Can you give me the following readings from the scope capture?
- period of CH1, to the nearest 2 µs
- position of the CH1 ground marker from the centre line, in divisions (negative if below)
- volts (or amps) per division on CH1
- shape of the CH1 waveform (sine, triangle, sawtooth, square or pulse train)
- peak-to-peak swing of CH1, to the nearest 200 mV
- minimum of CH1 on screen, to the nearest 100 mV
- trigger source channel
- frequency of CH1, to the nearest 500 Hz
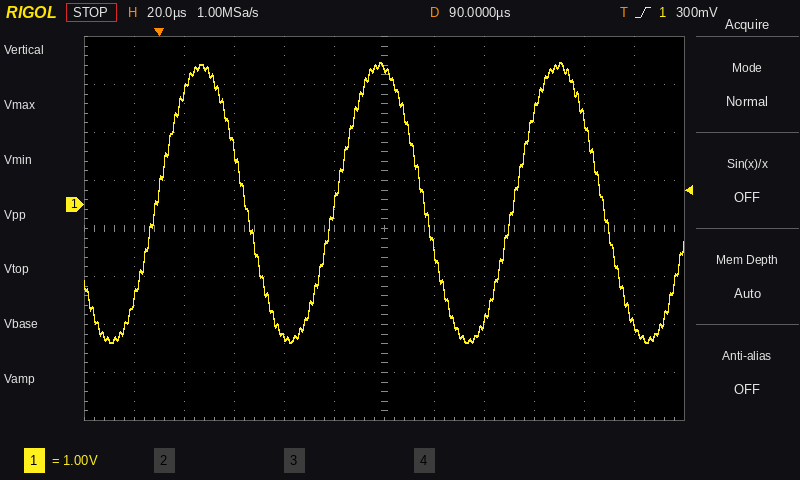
72 µs
+0.5 div
1 V
sine
5.8 V
-2.9 V
CH1
14.0 kHz
